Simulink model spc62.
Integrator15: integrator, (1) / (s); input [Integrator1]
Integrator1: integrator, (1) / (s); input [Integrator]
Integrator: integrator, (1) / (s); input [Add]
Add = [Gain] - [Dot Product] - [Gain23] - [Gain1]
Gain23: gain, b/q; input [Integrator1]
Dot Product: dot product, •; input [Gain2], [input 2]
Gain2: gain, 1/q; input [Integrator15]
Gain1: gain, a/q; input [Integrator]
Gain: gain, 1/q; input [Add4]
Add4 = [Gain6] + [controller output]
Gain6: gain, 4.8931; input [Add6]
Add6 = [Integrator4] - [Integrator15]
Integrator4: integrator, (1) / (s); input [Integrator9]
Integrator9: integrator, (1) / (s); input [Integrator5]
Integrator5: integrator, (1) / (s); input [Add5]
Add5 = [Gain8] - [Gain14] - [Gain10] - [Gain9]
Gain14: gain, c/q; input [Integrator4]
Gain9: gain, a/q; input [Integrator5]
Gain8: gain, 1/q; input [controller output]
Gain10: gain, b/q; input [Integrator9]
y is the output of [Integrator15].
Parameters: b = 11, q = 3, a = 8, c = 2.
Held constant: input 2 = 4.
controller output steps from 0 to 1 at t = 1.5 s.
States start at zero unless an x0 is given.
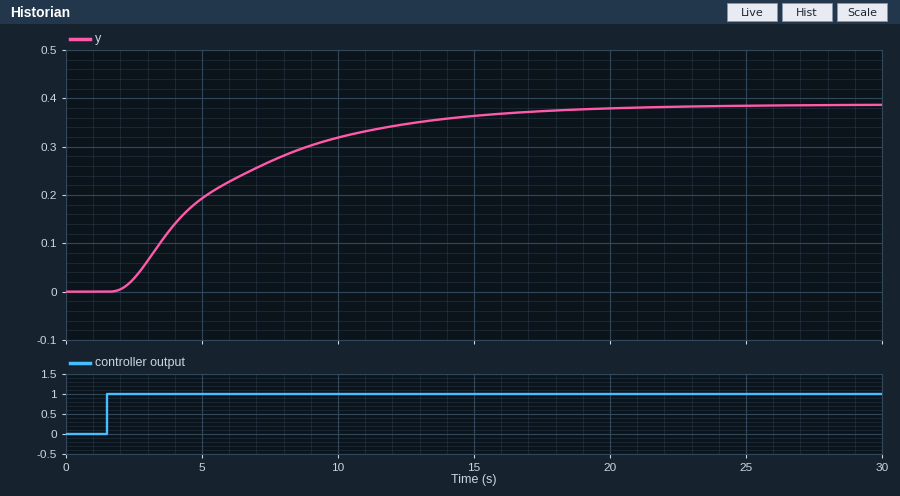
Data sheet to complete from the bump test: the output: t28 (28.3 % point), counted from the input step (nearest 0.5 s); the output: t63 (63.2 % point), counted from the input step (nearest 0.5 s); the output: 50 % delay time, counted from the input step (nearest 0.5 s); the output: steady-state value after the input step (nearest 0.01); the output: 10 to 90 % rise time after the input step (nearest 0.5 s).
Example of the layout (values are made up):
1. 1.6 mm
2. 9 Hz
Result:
1. 2.0 s
2. 5.0 s
3. 3.5 s
4. 0.39
5. 10.0 s
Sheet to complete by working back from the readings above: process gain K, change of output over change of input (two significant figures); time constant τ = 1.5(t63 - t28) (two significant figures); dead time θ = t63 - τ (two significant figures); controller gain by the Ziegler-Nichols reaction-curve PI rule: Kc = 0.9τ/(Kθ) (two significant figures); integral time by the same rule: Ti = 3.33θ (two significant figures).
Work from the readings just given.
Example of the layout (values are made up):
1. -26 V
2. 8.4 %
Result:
1. 0.39
2. 4.5 s
3. 0.50 s
4. 21
5. 1.7 s
